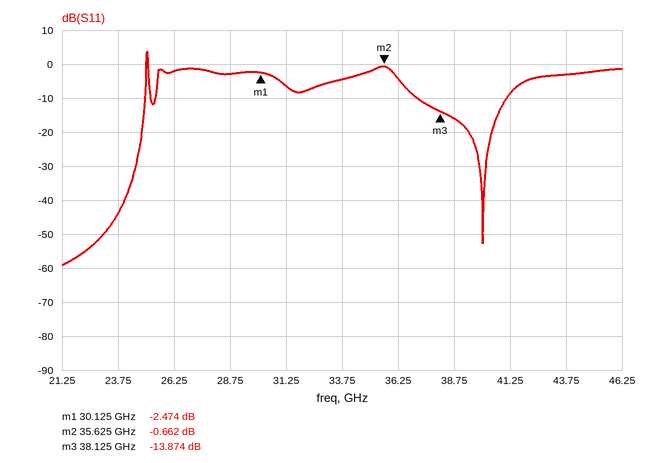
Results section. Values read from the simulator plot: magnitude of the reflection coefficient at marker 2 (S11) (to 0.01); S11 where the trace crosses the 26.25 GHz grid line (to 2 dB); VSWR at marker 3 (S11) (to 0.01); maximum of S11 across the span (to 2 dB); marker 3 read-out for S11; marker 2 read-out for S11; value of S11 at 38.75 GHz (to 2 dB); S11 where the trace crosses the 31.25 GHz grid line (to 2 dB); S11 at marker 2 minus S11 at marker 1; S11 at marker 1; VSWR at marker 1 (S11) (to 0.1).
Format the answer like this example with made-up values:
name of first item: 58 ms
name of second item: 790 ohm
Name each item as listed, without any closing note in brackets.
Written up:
magnitude of the reflection coefficient at marker 2 (S11): 0.93
S11 where the trace crosses the 26.25 GHz grid line: -2 dB
VSWR at marker 3 (S11): 1.51
maximum of S11 across the span: 4 dB
marker 3 read-out for S11: -13.874 dB
marker 2 read-out for S11: -0.662 dB
value of S11 at 38.75 GHz: -16 dB
S11 where the trace crosses the 31.25 GHz grid line: -6 dB
S11 at marker 2 minus S11 at marker 1: 1.812 dB
S11 at marker 1: -2.474 dB
VSWR at marker 1 (S11): 7.1
